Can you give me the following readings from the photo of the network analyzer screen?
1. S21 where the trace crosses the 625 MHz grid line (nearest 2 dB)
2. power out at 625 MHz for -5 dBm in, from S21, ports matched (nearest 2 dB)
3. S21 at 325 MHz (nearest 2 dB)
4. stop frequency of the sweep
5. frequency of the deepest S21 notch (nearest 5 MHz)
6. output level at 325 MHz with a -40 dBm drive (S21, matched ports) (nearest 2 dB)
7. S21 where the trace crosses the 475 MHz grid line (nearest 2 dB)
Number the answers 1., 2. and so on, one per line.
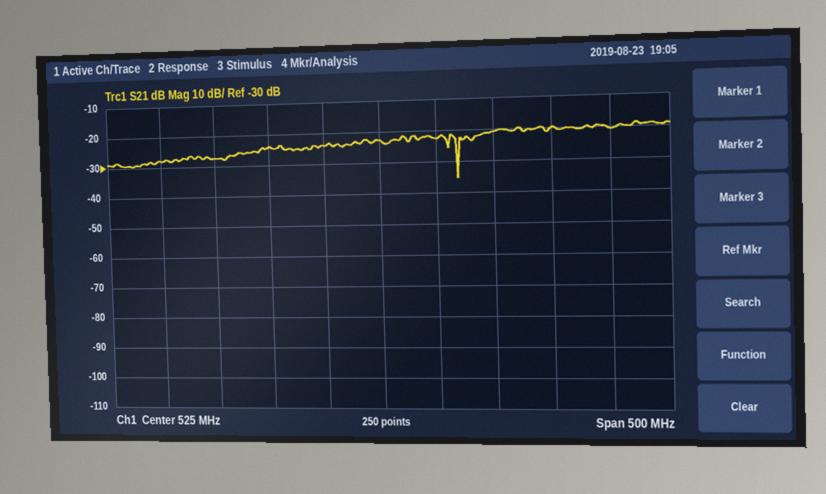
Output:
1. -20 dB
2. -26 dBm
3. -28 dB
4. 775 MHz
5. 595 MHz
6. -68 dBm
7. -24 dB
